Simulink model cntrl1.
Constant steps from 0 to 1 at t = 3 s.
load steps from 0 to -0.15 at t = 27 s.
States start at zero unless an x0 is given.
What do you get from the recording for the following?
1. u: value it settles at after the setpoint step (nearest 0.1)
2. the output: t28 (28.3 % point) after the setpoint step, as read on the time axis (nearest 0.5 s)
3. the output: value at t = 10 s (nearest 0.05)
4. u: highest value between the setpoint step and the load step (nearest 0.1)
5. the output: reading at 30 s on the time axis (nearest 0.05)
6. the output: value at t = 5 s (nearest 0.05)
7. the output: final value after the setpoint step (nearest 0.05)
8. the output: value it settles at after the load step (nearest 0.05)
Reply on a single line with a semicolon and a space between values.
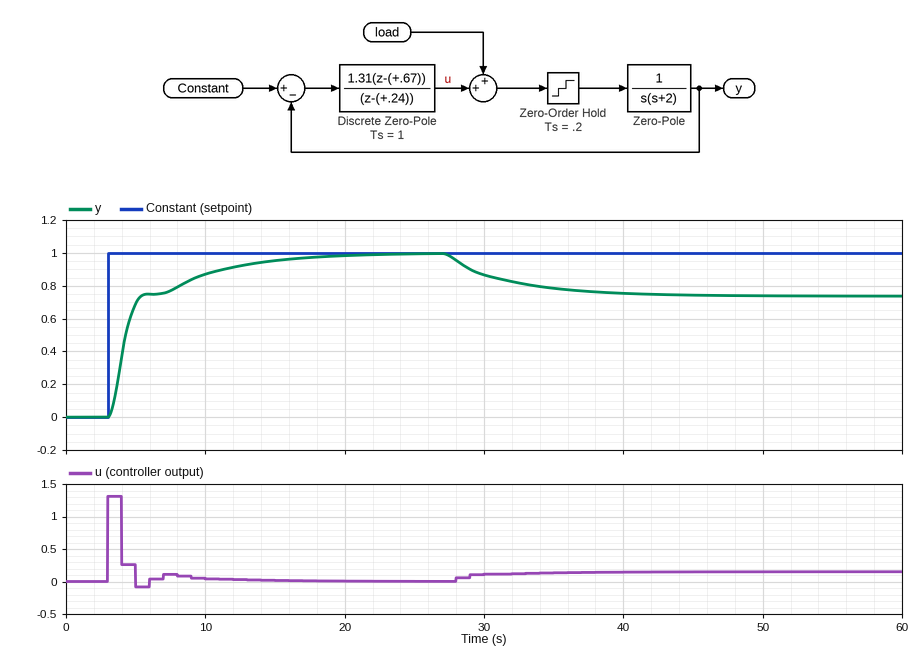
0.0; 4.0 s; 0.85; 1.3; 0.85; 0.70; 1.00; 0.75
